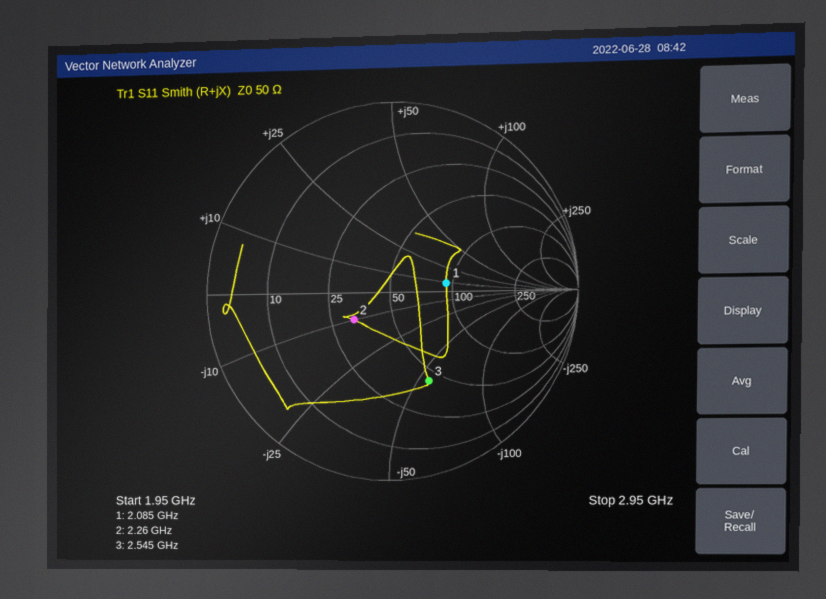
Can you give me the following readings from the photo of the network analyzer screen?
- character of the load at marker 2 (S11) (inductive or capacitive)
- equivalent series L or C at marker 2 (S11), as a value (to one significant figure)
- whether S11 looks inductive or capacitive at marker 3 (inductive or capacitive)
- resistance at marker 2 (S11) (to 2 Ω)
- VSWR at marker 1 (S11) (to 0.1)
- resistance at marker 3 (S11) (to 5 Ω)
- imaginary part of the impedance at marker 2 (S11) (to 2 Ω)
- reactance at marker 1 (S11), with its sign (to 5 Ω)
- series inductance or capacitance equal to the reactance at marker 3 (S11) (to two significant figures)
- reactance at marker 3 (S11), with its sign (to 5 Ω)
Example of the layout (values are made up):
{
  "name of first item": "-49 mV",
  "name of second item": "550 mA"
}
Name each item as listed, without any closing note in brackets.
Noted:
{
  "character of the load at marker 2 (S11)": "capacitive",
  "equivalent series L or C at marker 2 (S11), as a value": "7 pF",
  "whether S11 looks inductive or capacitive at marker 3": "capacitive",
  "resistance at marker 2 (S11)": "32 Ω",
  "VSWR at marker 1 (S11)": "1.9",
  "resistance at marker 3 (S11)": "45 Ω",
  "imaginary part of the impedance at marker 2 (S11)": "-10 Ω",
  "reactance at marker 1 (S11), with its sign": "+10 Ω",
  "series inductance or capacitance equal to the reactance at marker 3 (S11)": "1.1 pF",
  "reactance at marker 3 (S11), with its sign": "-55 Ω"
}
